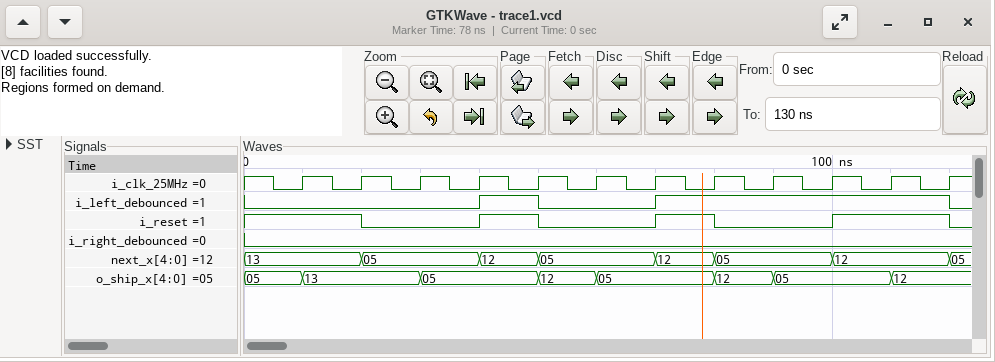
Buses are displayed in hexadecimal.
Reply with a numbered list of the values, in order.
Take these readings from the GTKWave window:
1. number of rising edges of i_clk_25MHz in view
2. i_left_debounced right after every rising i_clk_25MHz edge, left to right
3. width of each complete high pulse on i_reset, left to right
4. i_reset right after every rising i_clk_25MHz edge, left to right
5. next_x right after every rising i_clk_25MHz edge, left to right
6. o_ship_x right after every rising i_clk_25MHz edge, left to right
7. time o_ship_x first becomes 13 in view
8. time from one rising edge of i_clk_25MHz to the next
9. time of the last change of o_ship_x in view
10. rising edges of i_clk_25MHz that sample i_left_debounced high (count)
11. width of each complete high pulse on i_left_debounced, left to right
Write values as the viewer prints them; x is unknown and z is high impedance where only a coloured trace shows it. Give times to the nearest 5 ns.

1. 12
2. 0 0 0 1 0 0 1 1 1 1 1 0
3. 10 ns, 10 ns, 20 ns
4. 1 0 0 1 0 0 1 0 0 1 1 0
5. 13, 05, 05, 12, 05, 05, 12, 05, 05, 12, 12, 05
6. 13, 13, 05, 05, 12, 05, 05, 12, 05, 05, 12, 12
7. 10 ns
8. 10 ns
9. 110 ns
10. 6
11. 10 ns, 50 ns
